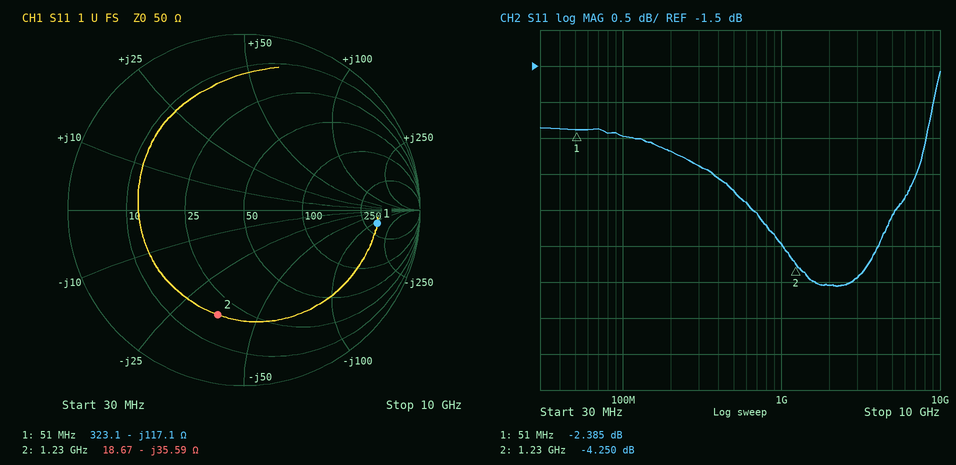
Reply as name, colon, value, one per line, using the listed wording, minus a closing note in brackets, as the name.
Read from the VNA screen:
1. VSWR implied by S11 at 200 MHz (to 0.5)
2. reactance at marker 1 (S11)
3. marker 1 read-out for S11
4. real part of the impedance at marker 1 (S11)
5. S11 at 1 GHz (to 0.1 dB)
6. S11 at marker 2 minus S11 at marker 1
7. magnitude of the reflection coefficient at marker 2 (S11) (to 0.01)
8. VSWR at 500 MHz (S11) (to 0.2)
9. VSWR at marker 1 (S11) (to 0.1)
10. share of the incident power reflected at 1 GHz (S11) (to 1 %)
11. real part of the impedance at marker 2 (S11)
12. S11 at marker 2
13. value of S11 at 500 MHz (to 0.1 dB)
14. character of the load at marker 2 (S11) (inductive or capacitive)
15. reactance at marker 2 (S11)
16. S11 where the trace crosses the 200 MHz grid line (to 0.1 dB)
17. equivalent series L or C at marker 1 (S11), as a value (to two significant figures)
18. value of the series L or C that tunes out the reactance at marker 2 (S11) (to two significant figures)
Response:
VSWR implied by S11 at 200 MHz: 6.5
reactance at marker 1: -117.1 Ω
marker 1 read-out for S11: -2.385 dB
real part of the impedance at marker 1: 323.1 Ω
S11 at 1 GHz: -4.0 dB
S11 at marker 2 minus S11 at marker 1: -1.865 dB
magnitude of the reflection coefficient at marker 2 (S11): 0.61
VSWR at 500 MHz (S11): 5.4
VSWR at marker 1 (S11): 7.3
share of the incident power reflected at 1 GHz (S11): 40 %
real part of the impedance at marker 2: 18.67 Ω
S11 at marker 2: -4.250 dB
value of S11 at 500 MHz: -3.2 dB
character of the load at marker 2 (S11): capacitive
reactance at marker 2: -35.59 Ω
S11 where the trace crosses the 200 MHz grid line: -2.7 dB
equivalent series L or C at marker 1 (S11), as a value: 27 pF
value of the series L or C that tunes out the reactance at marker 2 (S11): 4.6 nH
